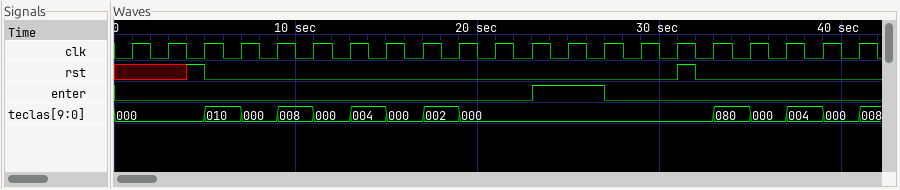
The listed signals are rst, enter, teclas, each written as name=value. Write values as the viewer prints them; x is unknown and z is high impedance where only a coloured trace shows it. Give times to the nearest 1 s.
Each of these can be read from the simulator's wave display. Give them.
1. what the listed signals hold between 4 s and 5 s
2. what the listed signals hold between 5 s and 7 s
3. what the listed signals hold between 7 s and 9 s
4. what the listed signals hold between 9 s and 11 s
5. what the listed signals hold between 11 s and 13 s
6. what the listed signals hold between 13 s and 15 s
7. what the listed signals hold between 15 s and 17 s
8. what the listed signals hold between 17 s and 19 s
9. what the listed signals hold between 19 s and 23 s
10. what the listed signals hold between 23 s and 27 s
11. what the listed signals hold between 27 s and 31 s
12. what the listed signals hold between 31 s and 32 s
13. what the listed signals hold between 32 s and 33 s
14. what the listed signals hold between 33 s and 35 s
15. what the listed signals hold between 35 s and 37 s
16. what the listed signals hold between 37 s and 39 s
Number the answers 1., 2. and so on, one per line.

1. rst=1, enter=0, teclas=000
2. rst=0, enter=0, teclas=010
3. rst=0, enter=0, teclas=000
4. rst=0, enter=0, teclas=008
5. rst=0, enter=0, teclas=000
6. rst=0, enter=0, teclas=004
7. rst=0, enter=0, teclas=000
8. rst=0, enter=0, teclas=002
9. rst=0, enter=0, teclas=000
10. rst=0, enter=1, teclas=000
11. rst=0, enter=0, teclas=000
12. rst=1, enter=0, teclas=000
13. rst=0, enter=0, teclas=000
14. rst=0, enter=0, teclas=080
15. rst=0, enter=0, teclas=000
16. rst=0, enter=0, teclas=004
